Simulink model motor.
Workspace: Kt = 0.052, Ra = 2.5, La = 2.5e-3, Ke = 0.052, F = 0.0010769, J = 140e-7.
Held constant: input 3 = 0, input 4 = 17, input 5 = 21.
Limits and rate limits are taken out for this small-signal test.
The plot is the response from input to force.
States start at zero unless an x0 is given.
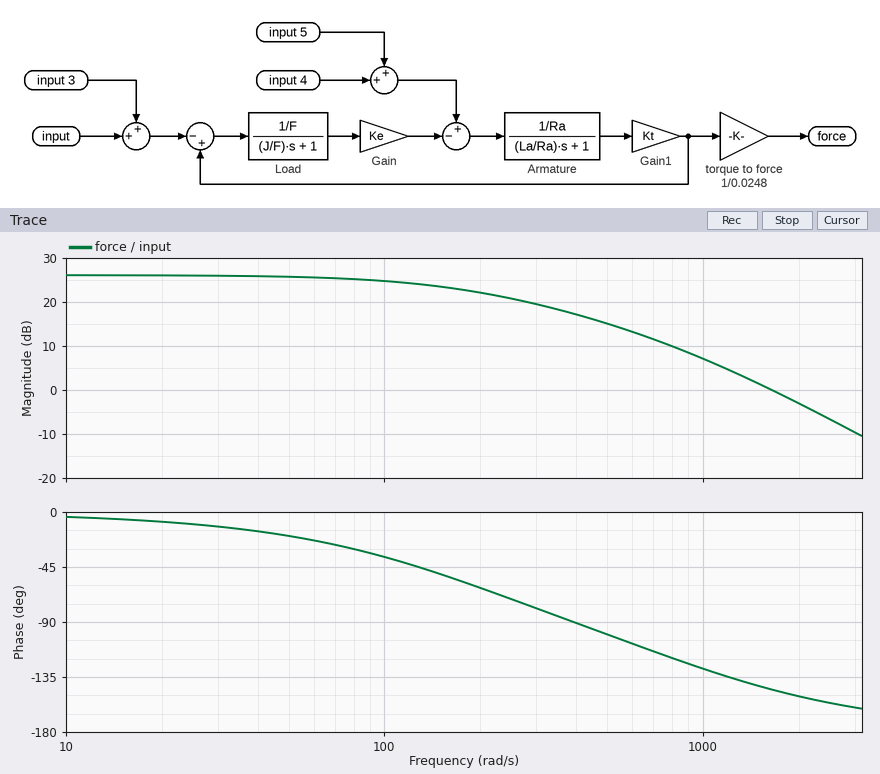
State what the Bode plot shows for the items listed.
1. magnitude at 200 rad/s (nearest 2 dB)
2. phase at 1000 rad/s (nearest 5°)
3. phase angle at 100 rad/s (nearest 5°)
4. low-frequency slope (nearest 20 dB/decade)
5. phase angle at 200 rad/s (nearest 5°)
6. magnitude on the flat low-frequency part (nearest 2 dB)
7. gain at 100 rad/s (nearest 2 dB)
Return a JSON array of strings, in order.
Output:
["22 dB", "-130°", "-35°", "0 dB/decade", "-60°", "26 dB", "24 dB"]
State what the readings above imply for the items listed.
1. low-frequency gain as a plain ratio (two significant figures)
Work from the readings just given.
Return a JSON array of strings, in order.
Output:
["20"]
